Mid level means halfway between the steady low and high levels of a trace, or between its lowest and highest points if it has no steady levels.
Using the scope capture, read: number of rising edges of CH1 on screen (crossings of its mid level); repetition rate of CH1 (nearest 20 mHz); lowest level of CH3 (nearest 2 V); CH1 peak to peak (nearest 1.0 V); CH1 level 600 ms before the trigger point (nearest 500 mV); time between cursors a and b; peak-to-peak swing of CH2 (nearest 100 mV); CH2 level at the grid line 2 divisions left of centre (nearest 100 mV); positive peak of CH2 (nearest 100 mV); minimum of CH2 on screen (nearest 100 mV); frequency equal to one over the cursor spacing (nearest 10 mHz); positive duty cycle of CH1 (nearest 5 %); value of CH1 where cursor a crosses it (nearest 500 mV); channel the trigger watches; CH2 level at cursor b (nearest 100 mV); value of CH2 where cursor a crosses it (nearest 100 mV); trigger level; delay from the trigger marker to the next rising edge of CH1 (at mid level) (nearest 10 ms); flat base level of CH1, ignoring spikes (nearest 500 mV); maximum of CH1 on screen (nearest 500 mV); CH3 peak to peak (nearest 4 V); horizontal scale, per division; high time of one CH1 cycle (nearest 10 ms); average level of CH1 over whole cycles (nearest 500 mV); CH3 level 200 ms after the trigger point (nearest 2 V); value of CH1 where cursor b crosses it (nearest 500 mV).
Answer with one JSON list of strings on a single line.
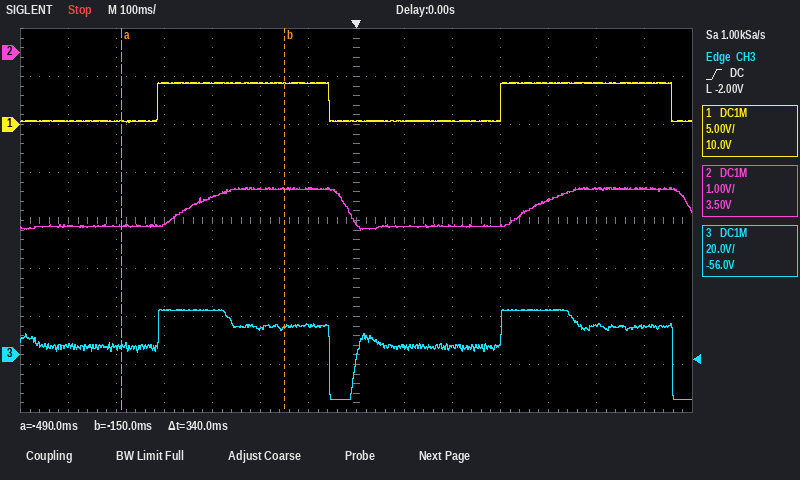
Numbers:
["2", "1.40 Hz", "-18 V", "4.0 V", "500 mV", "340 ms", "900 mV", "-2.8 V", "-2.8 V", "-3.7 V", "2.94 Hz", "50 %", "500 mV", "CH3", "-2.8 V", "-3.6 V", "-2.00 V", "300 ms", "500 mV", "4.5 V", "36 V", "100 ms", "360 ms", "2.5 V", "4 V", "4.5 V"]
